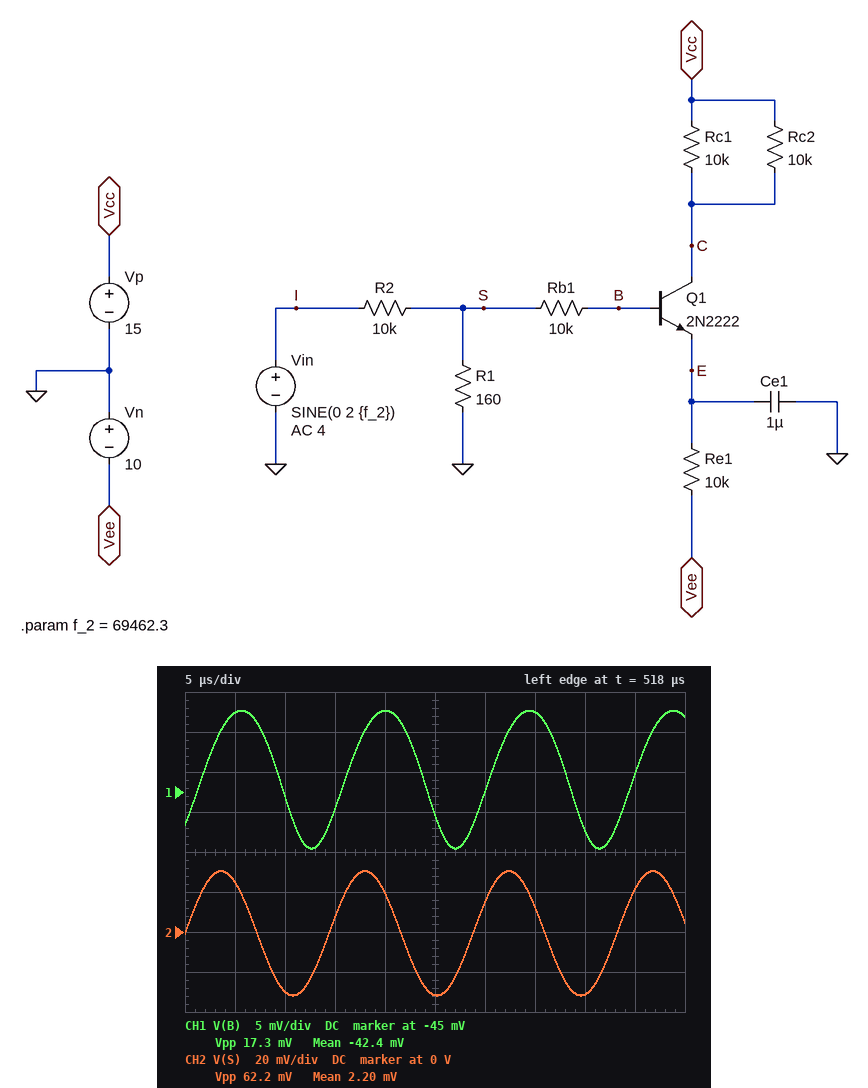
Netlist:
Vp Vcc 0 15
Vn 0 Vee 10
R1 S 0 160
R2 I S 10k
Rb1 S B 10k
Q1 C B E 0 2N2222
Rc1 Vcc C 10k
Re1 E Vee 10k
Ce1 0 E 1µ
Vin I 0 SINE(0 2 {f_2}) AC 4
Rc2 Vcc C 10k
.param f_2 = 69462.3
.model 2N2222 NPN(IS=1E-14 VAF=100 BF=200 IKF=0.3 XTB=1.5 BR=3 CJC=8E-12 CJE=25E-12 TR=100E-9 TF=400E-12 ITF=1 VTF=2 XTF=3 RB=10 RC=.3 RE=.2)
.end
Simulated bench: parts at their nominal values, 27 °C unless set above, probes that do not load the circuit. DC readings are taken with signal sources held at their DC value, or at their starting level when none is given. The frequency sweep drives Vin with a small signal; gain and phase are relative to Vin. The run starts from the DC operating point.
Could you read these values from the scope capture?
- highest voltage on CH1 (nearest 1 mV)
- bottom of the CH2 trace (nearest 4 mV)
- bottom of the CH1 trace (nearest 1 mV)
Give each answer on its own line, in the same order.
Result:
-35 mV
-32 mV
-52 mV
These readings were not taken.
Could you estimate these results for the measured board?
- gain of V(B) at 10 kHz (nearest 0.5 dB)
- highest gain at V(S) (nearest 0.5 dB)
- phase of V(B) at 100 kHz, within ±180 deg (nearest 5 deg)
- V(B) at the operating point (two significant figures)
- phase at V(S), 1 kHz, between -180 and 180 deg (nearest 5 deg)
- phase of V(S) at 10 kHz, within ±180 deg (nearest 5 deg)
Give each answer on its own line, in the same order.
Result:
-43.5 dB
-36.0 dB
-60 deg
-43 mV
0 deg
0 deg
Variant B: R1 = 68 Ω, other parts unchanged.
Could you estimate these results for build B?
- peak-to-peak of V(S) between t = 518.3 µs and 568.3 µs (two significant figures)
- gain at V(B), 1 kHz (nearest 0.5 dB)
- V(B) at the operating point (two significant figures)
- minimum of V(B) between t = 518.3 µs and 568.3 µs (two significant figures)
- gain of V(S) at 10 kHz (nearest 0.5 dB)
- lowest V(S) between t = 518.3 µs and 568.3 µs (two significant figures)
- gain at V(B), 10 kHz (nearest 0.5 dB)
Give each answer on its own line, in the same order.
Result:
27 mV
-44.0 dB
-42 mV
-46 mV
-43.5 dB
-14 mV
-50.5 dB
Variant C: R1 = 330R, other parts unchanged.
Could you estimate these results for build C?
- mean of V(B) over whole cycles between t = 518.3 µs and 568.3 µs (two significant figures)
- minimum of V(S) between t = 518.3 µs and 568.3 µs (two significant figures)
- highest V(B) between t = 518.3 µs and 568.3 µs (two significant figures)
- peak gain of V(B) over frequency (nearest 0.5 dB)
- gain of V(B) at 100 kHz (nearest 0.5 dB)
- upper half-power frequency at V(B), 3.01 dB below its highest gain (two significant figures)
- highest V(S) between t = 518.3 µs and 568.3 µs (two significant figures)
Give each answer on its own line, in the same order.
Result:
-44 mV
-64 mV
-28 mV
-30.0 dB
-43.5 dB
2.5 kHz
61 mV
